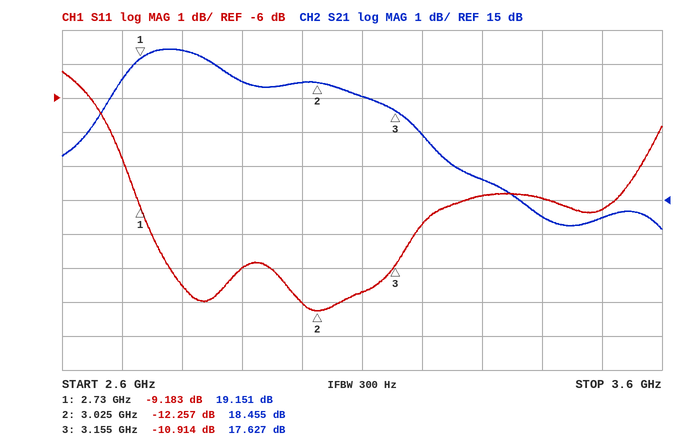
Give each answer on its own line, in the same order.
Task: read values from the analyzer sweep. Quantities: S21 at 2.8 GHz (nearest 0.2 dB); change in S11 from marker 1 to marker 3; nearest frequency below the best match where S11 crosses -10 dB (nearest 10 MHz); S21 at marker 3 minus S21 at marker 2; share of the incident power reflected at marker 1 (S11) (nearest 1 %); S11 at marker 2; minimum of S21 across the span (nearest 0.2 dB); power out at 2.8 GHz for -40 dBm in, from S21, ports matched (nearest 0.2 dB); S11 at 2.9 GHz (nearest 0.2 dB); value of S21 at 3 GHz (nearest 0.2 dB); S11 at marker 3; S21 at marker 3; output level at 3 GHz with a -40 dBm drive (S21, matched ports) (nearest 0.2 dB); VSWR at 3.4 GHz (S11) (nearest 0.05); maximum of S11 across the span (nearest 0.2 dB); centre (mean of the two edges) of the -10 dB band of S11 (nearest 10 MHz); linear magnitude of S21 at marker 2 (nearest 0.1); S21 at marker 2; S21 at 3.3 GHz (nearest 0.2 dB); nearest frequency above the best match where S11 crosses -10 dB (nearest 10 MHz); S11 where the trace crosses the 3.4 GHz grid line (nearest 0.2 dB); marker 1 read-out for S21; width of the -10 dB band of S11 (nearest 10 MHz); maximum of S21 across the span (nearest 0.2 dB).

19.4 dB
-1.731 dB
2.75 GHz
-0.828 dB
12 %
-12.257 dB
14.2 dB
-20.6 dBm
-11.0 dB
18.4 dB
-10.914 dB
17.627 dB
-21.6 dBm
2.10
-5.2 dB
2.97 GHz
8.4
18.455 dB
15.6 dB
3.19 GHz
-9.0 dB
19.151 dB
440 MHz
19.4 dB
